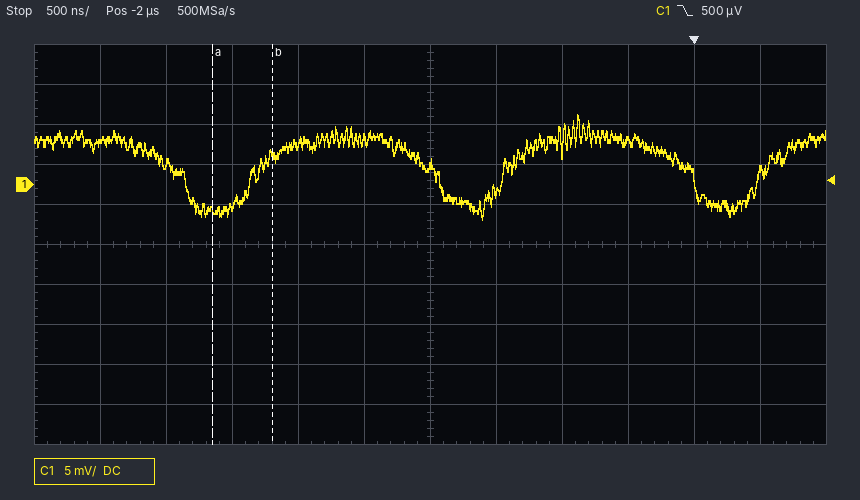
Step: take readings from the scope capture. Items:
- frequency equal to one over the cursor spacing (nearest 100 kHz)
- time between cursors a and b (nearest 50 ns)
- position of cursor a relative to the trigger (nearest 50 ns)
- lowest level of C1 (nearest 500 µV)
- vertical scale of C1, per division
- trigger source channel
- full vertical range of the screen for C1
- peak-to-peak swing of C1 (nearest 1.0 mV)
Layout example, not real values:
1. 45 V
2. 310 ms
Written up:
1. 2.2 MHz
2. 450 ns
3. -3.65 µs
4. -4.5 mV
5. 5 mV
6. C1
7. 50 mV
8. 13.0 mV
